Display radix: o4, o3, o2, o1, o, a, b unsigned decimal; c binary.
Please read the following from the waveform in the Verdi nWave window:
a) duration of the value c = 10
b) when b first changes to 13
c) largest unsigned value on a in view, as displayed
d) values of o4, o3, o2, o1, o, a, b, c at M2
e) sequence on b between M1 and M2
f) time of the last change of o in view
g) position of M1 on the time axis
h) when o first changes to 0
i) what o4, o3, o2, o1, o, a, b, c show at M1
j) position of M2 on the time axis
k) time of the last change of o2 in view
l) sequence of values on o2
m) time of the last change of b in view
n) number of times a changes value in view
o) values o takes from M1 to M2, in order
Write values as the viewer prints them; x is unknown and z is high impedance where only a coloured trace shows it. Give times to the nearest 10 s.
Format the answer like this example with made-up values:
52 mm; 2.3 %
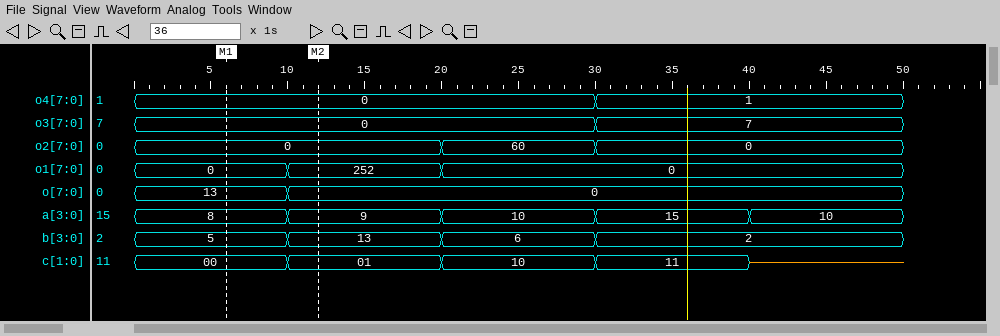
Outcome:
10 s; 10 s; 15; o4=0, o3=0, o2=0, o1=252, o=0, a=9, b=13, c=01; 5, 13; 10 s; 10 s; 10 s; o4=0, o3=0, o2=0, o1=0, o=13, a=8, b=5, c=00; 10 s; 30 s; 0, 60, 0; 30 s; 4; 13, 0
